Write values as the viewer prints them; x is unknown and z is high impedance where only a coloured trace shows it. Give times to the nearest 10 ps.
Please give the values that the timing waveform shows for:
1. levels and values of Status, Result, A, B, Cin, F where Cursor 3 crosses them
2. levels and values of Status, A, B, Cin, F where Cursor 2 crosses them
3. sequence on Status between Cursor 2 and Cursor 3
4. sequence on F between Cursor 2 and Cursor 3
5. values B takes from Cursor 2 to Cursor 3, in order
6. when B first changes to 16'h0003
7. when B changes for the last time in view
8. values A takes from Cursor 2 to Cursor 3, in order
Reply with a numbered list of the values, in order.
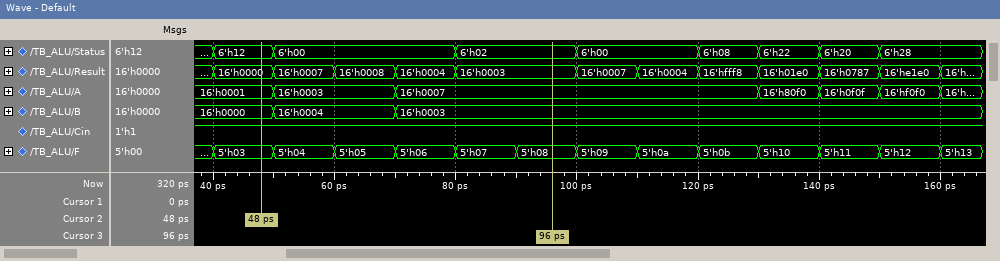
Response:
1. Status=6'h02, Result=16'h0003, A=16'h0007, B=16'h0003, Cin=1, F=5'h08
2. Status=6'h12, A=16'h0001, B=16'h0000, Cin=1, F=5'h03
3. 6'h12, 6'h00, 6'h02
4. 5'h03, 5'h04, 5'h05, 5'h06, 5'h07, 5'h08
5. 16'h0000, 16'h0004, 16'h0003
6. 70 ps
7. 70 ps
8. 16'h0001, 16'h0003, 16'h0007
